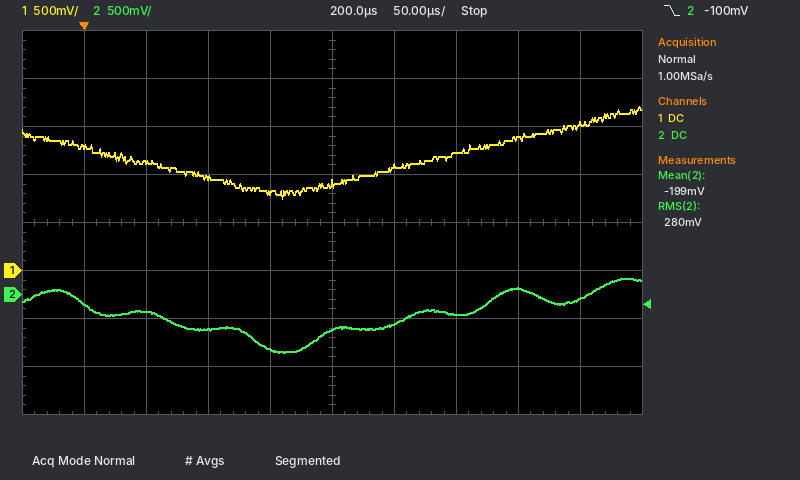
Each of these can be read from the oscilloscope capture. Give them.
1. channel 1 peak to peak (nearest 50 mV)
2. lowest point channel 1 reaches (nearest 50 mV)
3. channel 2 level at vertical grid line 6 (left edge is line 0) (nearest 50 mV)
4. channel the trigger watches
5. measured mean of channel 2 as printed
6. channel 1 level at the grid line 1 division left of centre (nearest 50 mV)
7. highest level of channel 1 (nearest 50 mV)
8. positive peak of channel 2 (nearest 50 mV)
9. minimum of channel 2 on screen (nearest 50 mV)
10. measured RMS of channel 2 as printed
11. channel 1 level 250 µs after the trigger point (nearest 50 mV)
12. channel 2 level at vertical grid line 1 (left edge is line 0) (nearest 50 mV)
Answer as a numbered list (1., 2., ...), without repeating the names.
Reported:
1. 950 mV
2. 750 mV
3. -300 mV
4. channel 2
5. -199 mV
6. 800 mV
7. 1.70 V
8. 150 mV
9. -600 mV
10. 280 mV
11. 1.10 V
12. -100 mV
